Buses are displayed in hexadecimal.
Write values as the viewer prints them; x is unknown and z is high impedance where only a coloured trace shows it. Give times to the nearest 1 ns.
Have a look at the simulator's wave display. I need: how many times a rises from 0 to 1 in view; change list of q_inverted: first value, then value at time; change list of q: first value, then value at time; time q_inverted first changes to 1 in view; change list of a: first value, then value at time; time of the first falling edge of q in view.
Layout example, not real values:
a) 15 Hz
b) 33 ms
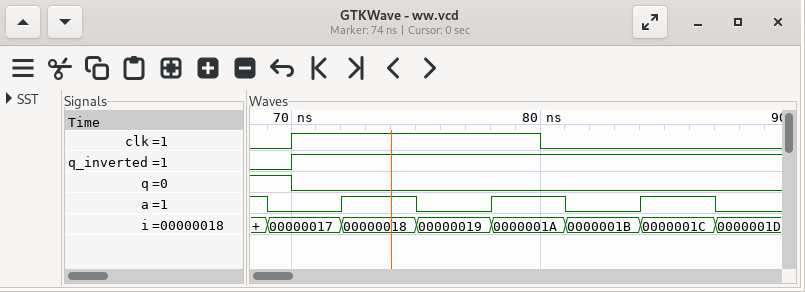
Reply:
a) 3
b) 0, 1 at 70 ns
c) 1, 0 at 70 ns
d) 70 ns
e) 1, 0 at 69 ns, 1 at 72 ns, 0 at 75 ns, 1 at 78 ns, 0 at 81 ns, 1 at 84 ns, 0 at 87 ns
f) 70 ns
